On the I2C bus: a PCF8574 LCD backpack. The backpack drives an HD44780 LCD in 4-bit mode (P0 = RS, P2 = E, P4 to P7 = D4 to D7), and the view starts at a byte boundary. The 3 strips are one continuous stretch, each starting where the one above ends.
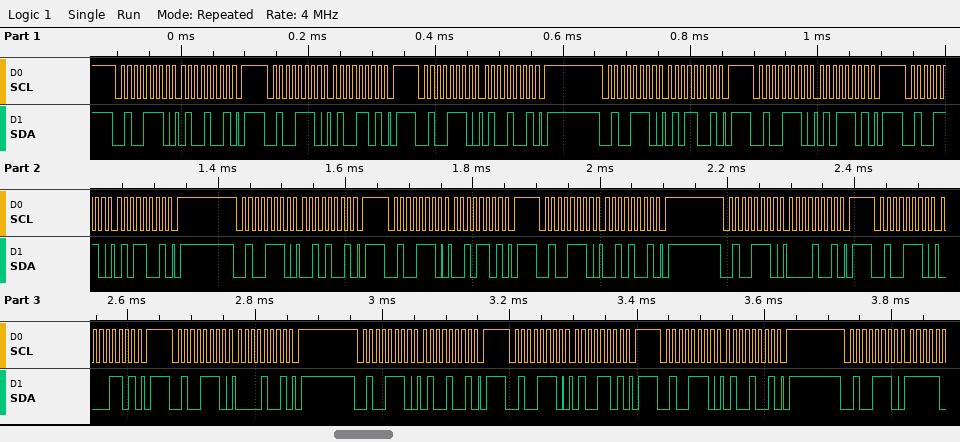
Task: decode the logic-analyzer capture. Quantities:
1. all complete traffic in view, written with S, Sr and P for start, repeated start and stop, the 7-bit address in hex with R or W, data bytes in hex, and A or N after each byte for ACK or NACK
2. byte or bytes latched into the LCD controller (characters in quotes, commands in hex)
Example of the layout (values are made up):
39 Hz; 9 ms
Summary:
S 27W A 49 A P S 27W A 4D A P S 27W A 49 A P S 27W A 59 A P S 27W A 5D A P S 27W A 59 A P S 27W A 29 A P S 27W A 2D A P S 27W A 29 A P S 27W A 09 A P S 27W A 0D A P S 27W A 09 A P S 27W A 49 A P S 27W A 4D A P S 27W A 49 A P S 27W A; 'E' ' '
